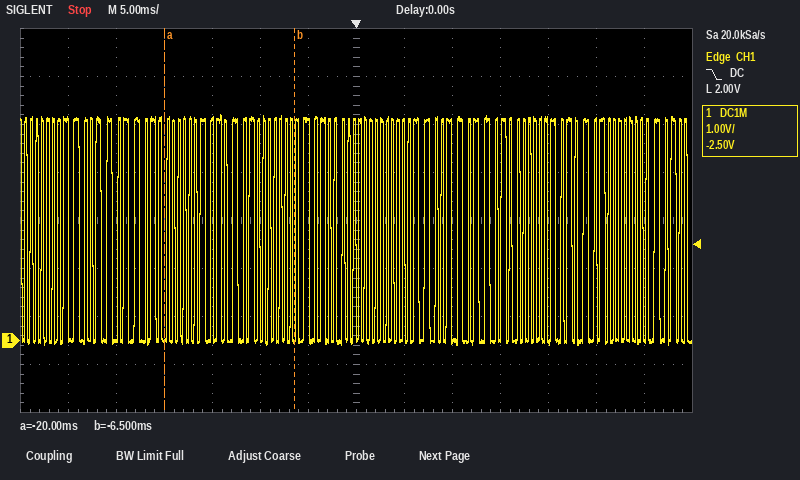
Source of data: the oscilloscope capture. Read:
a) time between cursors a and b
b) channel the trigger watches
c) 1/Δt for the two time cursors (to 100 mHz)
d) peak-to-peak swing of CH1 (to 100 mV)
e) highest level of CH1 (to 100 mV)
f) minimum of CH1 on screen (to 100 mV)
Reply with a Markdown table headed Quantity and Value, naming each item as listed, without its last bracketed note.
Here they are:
| Quantity | Value |
|---|---|
| time between cursors a and b | 13.5 ms |
| channel the trigger watches | CH1 |
| 1/Δt for the two time cursors | 74.1 Hz |
| peak-to-peak swing of CH1 | 4.8 V |
| highest level of CH1 | 4.7 V |
| minimum of CH1 on screen | -100 mV |
